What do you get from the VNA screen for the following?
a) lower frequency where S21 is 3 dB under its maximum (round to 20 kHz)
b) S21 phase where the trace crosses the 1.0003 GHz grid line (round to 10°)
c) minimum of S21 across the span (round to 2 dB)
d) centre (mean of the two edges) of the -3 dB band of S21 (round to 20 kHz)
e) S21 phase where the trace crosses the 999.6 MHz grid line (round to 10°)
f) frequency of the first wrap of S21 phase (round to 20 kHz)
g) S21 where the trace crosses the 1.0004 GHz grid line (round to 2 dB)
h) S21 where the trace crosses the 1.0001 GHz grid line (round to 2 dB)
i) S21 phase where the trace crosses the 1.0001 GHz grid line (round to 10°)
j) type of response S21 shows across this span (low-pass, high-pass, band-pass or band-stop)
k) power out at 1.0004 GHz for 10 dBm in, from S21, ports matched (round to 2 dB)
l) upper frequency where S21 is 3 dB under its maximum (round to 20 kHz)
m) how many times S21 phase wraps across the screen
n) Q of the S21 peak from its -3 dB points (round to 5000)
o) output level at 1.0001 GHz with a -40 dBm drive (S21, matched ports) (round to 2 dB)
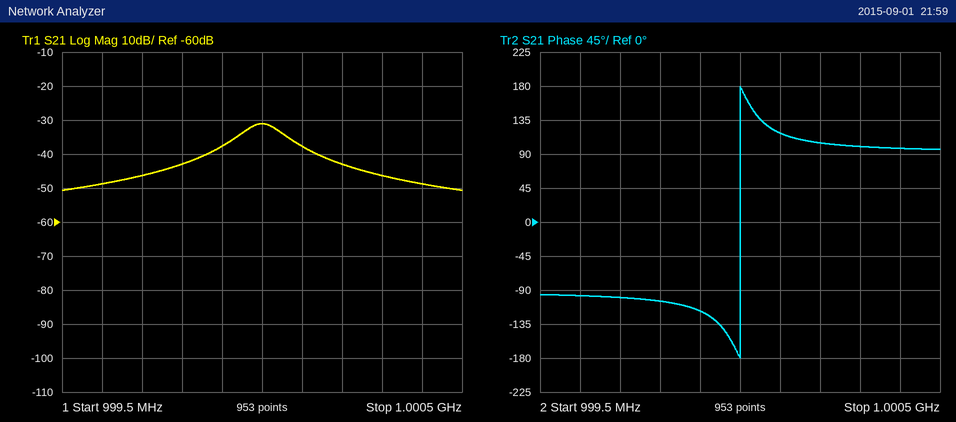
999.94 MHz
100°
-50 dB
1.00000 GHz
-100°
1.00000 GHz
-48 dB
-38 dB
120°
band-pass
-38 dBm
1.00006 GHz
1
10000
-78 dBm
